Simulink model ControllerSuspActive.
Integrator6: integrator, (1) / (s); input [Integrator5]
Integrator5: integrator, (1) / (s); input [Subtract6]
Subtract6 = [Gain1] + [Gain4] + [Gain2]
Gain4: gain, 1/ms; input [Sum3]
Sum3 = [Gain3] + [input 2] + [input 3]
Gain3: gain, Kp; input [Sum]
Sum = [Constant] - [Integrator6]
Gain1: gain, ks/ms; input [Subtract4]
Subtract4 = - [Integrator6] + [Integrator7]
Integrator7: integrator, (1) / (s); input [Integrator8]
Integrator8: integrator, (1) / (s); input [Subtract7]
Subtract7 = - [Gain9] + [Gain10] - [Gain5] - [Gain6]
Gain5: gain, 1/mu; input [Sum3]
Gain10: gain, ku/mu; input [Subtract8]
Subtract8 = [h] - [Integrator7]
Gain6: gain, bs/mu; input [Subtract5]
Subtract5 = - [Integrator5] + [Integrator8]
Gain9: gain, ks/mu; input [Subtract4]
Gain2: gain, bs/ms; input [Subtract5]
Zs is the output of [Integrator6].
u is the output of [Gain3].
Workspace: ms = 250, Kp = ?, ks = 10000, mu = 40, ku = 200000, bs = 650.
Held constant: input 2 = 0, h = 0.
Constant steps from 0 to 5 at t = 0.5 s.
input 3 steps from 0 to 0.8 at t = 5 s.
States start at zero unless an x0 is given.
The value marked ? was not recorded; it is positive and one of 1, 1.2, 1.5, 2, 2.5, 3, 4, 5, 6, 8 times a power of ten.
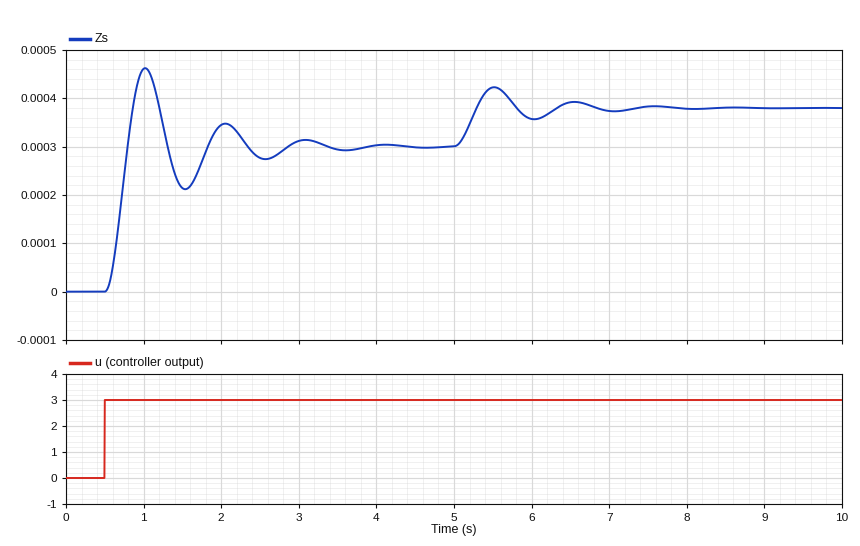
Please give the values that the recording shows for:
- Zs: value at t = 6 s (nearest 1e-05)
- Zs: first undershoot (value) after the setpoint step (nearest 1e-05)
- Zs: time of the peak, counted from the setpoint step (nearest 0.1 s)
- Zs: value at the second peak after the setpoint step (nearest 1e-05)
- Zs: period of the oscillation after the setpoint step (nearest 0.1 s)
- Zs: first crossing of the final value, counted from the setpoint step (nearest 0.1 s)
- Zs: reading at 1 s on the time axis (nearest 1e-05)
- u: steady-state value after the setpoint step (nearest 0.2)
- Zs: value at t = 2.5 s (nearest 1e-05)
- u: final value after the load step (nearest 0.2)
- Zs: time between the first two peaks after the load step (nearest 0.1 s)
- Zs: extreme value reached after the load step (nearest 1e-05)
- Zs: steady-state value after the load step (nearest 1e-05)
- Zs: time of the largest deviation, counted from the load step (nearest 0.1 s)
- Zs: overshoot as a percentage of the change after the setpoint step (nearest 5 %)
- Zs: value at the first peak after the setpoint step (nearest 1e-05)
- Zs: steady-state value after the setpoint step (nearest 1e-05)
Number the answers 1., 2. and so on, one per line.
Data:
1. 0.00036
2. 0.00021
3. 0.5 s
4. 0.00035
5. 1.0 s
6. 0.3 s
7. 0.00046
8. 3.0
9. 0.00028
10. 3.0
11. 1.0 s
12. 0.00042
13. 0.00038
14. 0.5 s
15. 55 %
16. 0.00046
17. 0.00030
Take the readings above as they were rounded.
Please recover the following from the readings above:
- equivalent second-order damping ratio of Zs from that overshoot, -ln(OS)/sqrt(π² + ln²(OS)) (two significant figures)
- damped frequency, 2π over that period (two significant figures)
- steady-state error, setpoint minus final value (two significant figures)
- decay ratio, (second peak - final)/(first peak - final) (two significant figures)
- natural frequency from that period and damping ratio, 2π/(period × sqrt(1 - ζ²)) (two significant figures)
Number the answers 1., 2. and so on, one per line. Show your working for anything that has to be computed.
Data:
1. ln(0.55) = -0.598; 0.598 / sqrt(9.870 + 0.357) = 0.19
2. 2π / 1 = 6.3 rad/s
3. 5 - 0.0003 = 5.0
4. (0.00035 - 0.0003) / (0.00046 - 0.0003) = 0.31
5. 2π / (1 × sqrt(1 - 0.19²)) = 6.4 rad/s
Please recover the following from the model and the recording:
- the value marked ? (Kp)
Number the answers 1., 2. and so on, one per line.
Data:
1. 0.6
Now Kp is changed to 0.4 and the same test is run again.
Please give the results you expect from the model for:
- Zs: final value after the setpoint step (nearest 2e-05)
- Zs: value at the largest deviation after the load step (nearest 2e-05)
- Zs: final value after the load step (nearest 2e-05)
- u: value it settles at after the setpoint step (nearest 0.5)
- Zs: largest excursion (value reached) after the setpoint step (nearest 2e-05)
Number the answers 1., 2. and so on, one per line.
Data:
1. 0.00020
2. 0.00032
3. 0.00028
4. 2.0
5. 0.00030
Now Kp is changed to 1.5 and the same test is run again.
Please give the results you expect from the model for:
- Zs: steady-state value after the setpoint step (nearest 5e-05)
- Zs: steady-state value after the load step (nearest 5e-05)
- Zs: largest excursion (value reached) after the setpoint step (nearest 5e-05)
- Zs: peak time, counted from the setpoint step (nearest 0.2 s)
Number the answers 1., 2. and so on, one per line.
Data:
1. 0.00075
2. 0.00085
3. 0.00115
4. 0.6 s
